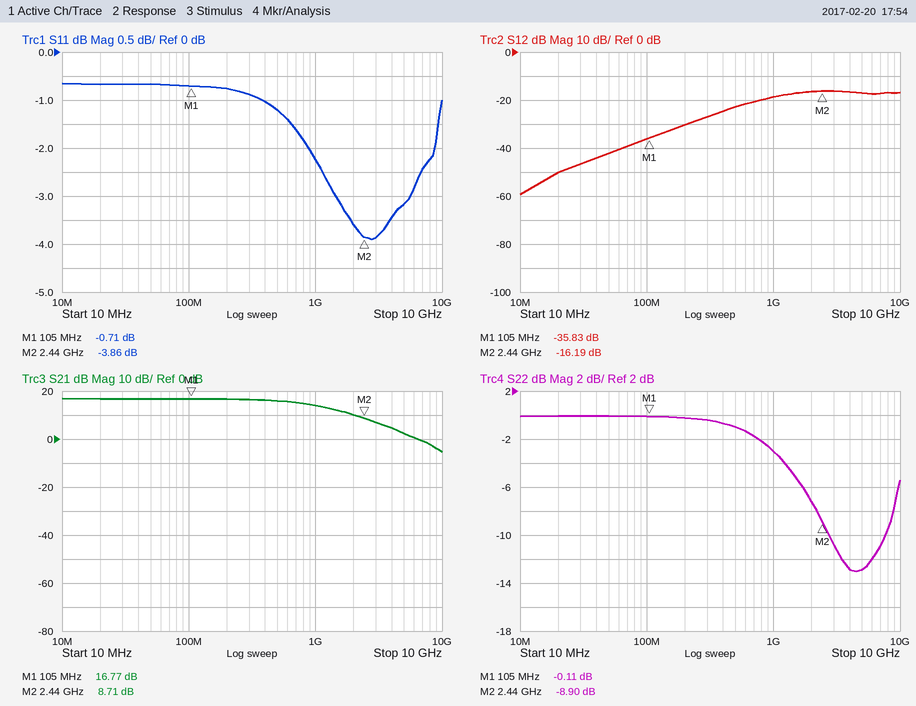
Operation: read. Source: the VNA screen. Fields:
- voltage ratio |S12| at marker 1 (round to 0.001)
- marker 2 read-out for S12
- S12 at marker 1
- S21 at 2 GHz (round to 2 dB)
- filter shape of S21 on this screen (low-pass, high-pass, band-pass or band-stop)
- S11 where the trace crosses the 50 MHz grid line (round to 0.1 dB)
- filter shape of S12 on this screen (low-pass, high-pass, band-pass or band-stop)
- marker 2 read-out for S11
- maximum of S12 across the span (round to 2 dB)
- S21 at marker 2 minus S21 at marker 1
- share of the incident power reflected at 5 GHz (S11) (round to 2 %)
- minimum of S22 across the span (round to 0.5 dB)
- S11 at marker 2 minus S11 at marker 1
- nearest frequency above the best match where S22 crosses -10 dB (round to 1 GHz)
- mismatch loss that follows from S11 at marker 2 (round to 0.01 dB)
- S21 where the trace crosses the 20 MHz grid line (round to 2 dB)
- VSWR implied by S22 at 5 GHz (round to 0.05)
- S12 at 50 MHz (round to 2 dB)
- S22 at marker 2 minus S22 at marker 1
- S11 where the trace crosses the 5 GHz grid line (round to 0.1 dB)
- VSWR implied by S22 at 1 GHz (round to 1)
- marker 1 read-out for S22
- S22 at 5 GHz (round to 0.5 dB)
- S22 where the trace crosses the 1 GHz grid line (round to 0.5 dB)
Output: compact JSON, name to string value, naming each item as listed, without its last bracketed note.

{"voltage ratio |S12| at marker 1": "0.016", "marker 2 read-out for S12": "-16.19 dB", "S12 at marker 1": "-35.83 dB", "S21 at 2 GHz": "10 dB", "filter shape of S21 on this screen": "low-pass", "S11 where the trace crosses the 50 MHz grid line": "-0.7 dB", "filter shape of S12 on this screen": "high-pass", "marker 2 read-out for S11": "-3.86 dB", "maximum of S12 across the span": "-16 dB", "S21 at marker 2 minus S21 at marker 1": "-8.06 dB", "share of the incident power reflected at 5 GHz (S11)": "48 %", "minimum of S22 across the span": "-13.0 dB", "S11 at marker 2 minus S11 at marker 1": "-3.15 dB", "nearest frequency above the best match where S22 crosses -10 dB": "8 GHz", "mismatch loss that follows from S11 at marker 2": "2.30 dB", "S21 where the trace crosses the 20 MHz grid line": "16 dB", "VSWR implied by S22 at 5 GHz": "1.60", "S12 at 50 MHz": "-42 dB", "S22 at marker 2 minus S22 at marker 1": "-8.79 dB", "S11 where the trace crosses the 5 GHz grid line": "-3.2 dB", "VSWR implied by S22 at 1 GHz": "6", "marker 1 read-out for S22": "-0.11 dB", "S22 at 5 GHz": "-13.0 dB", "S22 where the trace crosses the 1 GHz grid line": "-3.0 dB"}
